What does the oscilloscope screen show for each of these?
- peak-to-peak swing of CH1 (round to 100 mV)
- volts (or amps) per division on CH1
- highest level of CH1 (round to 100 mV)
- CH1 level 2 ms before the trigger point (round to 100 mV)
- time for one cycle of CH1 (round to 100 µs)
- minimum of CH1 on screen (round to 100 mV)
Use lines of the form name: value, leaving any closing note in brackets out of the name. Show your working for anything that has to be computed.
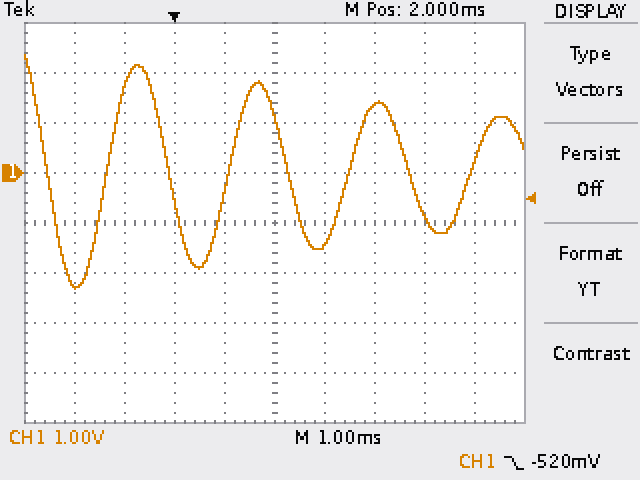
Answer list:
peak-to-peak swing of CH1: 2.4 V − (-2.3 V) = 4.7 V
volts (or amps) per division on CH1: 1 V
highest level of CH1: 2.4 V
CH1 level 2 ms before the trigger point: -2.2 V
time for one cycle of CH1: 2.4 ms
minimum of CH1 on screen: -2.3 V
